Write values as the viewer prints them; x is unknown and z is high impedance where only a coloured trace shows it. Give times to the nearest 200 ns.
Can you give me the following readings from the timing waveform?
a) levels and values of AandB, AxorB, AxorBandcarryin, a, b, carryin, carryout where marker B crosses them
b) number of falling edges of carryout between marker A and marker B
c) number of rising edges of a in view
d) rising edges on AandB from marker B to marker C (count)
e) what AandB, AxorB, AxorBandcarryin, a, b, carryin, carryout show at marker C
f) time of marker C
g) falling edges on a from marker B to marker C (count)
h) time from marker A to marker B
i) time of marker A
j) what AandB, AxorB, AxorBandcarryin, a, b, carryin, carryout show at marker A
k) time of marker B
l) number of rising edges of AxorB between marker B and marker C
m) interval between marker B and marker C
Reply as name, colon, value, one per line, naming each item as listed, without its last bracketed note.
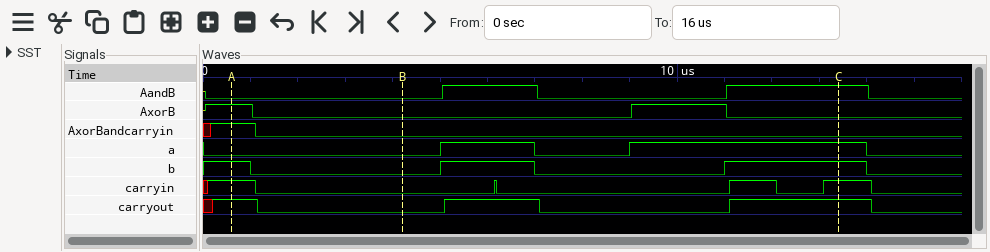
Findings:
levels and values of AandB, AxorB, AxorBandcarryin, a, b, carryin, carryout where marker B crosses them: AandB=0, AxorB=0, AxorBandcarryin=0, a=0, b=0, carryin=0, carryout=0
number of falling edges of carryout between marker A and marker B: 1
number of rising edges of a in view: 2
rising edges on AandB from marker B to marker C: 2
what AandB, AxorB, AxorBandcarryin, a, b, carryin, carryout show at marker C: AandB=1, AxorB=0, AxorBandcarryin=0, a=1, b=1, carryin=1, carryout=1
time of marker C: 13400 ns
falling edges on a from marker B to marker C: 1
time from marker A to marker B: 3600 ns
time of marker A: 600 ns
what AandB, AxorB, AxorBandcarryin, a, b, carryin, carryout show at marker A: AandB=0, AxorB=1, AxorBandcarryin=1, a=0, b=1, carryin=1, carryout=1
time of marker B: 4200 ns
number of rising edges of AxorB between marker B and marker C: 1
interval between marker B and marker C: 9200 ns
